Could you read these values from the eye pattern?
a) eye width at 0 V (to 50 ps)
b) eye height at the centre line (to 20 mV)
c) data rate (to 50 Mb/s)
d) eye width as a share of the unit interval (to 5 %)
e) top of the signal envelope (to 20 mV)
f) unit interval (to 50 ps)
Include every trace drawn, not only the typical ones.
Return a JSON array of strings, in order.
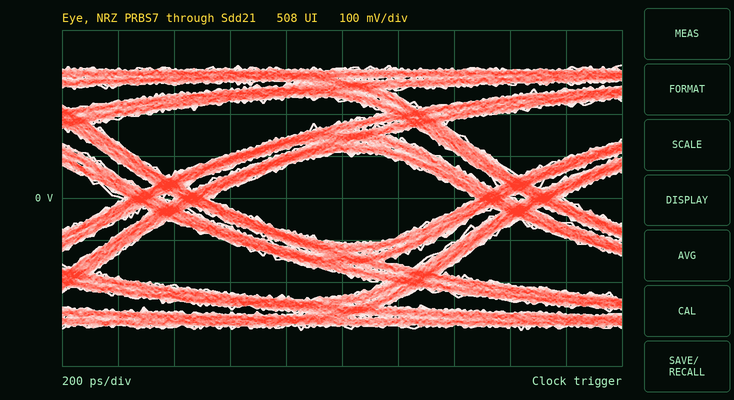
["950 ps", "220 mV", "800 Mb/s", "75 %", "320 mV", "1.25 ns"]
